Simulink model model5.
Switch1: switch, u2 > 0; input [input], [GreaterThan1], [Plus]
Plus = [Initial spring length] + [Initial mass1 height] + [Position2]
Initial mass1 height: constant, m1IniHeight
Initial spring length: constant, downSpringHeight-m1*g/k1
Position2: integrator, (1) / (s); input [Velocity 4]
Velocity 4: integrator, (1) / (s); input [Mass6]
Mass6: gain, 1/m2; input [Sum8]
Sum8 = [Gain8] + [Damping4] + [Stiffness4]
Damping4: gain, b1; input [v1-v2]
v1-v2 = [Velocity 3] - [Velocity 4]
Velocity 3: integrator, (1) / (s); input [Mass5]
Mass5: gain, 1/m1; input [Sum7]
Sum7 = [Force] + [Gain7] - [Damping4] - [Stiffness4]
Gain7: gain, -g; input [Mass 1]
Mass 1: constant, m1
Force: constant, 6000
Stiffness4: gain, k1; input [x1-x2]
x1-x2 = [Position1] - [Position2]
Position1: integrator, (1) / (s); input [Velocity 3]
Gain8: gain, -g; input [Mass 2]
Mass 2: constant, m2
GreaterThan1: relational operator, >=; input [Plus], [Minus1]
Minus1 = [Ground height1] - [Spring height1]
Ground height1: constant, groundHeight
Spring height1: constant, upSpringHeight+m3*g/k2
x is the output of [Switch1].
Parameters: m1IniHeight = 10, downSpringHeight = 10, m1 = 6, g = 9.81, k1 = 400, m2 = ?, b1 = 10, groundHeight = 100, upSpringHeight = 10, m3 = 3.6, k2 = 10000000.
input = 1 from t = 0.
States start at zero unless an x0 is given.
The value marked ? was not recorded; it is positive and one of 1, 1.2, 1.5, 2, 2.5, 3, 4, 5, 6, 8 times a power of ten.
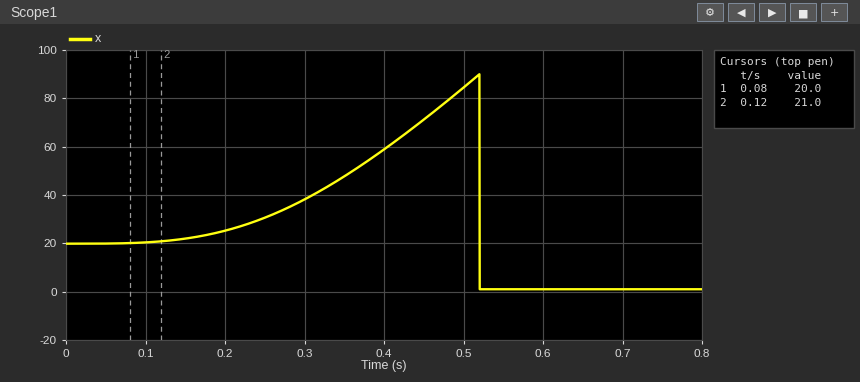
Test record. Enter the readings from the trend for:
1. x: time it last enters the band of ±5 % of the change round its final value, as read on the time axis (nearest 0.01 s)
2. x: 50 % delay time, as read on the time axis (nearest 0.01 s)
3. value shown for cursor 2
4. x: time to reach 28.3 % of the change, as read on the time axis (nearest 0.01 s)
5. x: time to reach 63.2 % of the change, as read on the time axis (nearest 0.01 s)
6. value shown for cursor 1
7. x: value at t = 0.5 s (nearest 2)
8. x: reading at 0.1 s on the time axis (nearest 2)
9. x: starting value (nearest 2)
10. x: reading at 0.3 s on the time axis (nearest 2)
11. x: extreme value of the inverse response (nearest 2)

0.52 s
0.52 s
21.0
0.52 s
0.52 s
20.0
84
20
20
38
90
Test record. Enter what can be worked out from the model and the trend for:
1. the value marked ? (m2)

5
